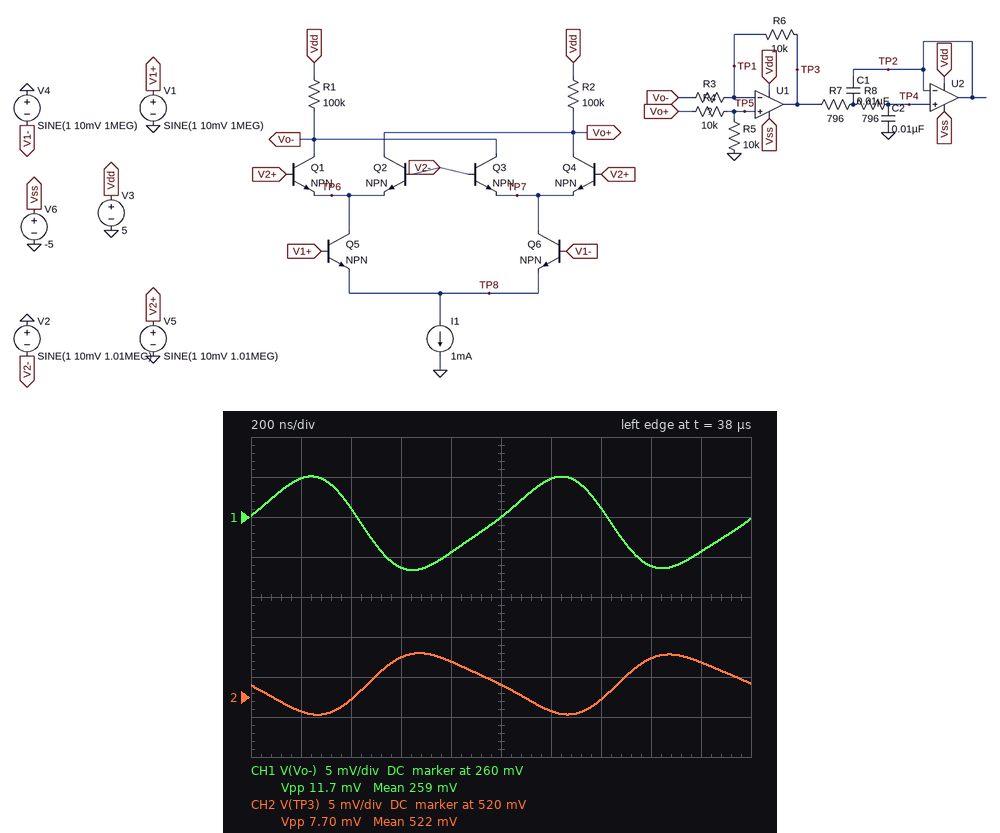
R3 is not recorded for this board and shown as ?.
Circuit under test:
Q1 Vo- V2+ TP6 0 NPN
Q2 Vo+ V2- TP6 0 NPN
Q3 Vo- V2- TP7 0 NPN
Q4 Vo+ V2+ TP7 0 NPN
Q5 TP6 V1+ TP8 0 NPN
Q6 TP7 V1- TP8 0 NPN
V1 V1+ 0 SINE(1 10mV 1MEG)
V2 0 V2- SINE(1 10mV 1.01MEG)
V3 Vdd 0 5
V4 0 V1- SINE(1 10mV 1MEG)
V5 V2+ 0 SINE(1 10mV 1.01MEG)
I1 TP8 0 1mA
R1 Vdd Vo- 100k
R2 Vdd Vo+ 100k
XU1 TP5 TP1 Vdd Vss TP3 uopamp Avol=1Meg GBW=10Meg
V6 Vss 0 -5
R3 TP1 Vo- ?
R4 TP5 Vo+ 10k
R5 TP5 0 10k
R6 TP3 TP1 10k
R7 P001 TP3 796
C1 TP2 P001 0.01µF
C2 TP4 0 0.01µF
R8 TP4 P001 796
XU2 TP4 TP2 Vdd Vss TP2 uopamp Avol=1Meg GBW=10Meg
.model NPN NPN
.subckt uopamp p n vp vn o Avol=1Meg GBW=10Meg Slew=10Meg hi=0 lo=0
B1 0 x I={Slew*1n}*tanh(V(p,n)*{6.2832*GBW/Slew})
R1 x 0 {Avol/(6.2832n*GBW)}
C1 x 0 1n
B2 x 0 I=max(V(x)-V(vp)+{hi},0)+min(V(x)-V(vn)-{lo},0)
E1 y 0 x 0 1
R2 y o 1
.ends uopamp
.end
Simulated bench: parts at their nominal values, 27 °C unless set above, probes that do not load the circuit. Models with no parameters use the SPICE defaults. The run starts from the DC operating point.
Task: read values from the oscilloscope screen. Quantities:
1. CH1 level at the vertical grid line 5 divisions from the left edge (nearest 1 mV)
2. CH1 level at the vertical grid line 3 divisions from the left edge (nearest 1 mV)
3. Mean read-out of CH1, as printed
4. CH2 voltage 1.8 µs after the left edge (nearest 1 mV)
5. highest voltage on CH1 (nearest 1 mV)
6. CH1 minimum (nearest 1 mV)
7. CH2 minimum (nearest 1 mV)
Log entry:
260 mV
254 mV
259 mV
524 mV
265 mV
253 mV
518 mV
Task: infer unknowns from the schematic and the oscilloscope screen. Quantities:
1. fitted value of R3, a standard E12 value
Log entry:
15 kΩ
